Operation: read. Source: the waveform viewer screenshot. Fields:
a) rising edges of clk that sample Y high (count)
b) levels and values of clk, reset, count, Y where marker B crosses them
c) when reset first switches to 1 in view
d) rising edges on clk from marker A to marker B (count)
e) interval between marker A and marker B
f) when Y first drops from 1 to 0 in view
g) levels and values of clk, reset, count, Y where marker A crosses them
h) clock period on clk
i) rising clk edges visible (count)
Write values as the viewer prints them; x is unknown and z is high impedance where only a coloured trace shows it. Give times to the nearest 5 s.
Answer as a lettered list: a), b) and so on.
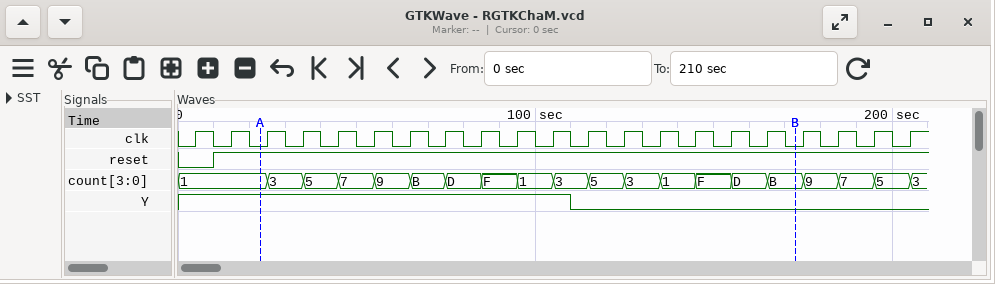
a) 11
b) clk=0, reset=1, count=B, Y=0
c) 10 s
d) 15
e) 150 s
f) 110 s
g) clk=0, reset=1, count=1, Y=1
h) 10 s
i) 21
